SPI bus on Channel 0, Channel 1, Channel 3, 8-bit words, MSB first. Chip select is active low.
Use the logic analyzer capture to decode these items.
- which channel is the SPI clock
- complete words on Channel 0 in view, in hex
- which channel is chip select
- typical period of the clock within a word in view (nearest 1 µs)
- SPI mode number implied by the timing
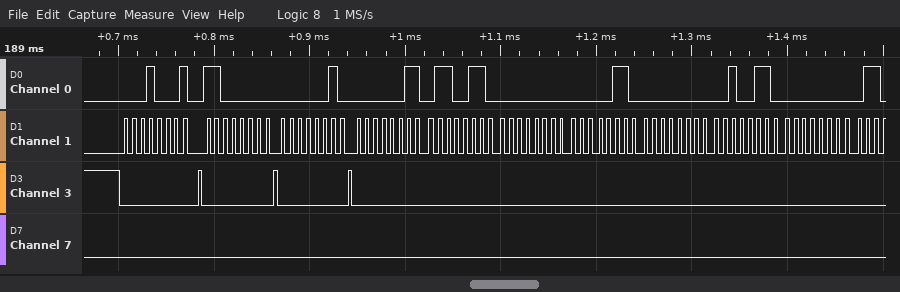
Channel 1
11, C0, 02, 03, 66, 00, 06, 00, 26, 00
Channel 3
9 µs
0
